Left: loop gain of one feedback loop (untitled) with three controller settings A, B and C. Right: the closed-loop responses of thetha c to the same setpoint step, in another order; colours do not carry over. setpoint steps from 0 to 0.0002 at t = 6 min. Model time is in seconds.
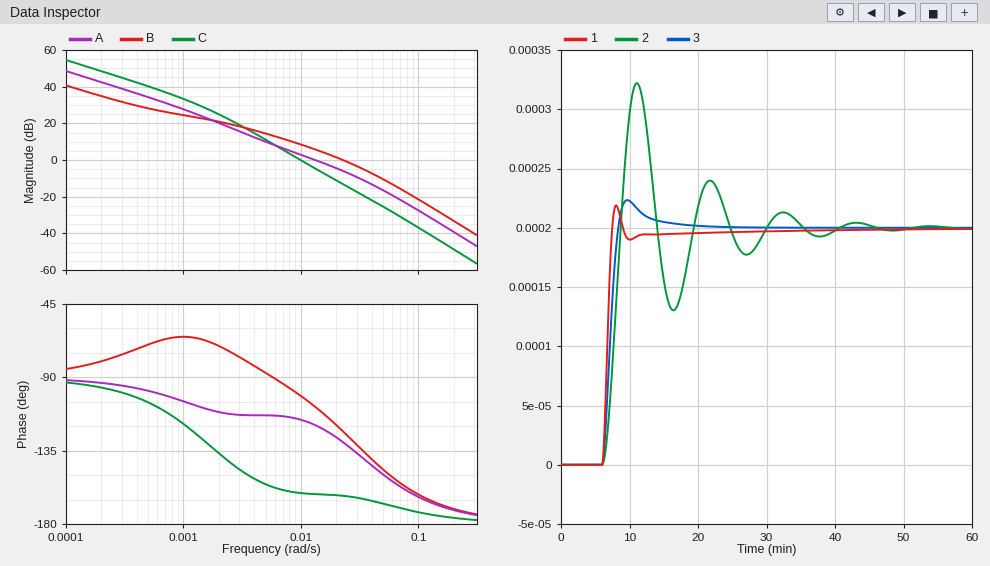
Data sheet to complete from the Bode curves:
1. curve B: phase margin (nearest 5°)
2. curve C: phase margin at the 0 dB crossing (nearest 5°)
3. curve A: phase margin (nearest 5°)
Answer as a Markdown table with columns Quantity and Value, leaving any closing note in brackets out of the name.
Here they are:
| Quantity | Value |
|---|---|
| curve B: phase margin | 55° |
| curve C: phase margin at the 0 dB crossing | 20° |
| curve A: phase margin | 60° |
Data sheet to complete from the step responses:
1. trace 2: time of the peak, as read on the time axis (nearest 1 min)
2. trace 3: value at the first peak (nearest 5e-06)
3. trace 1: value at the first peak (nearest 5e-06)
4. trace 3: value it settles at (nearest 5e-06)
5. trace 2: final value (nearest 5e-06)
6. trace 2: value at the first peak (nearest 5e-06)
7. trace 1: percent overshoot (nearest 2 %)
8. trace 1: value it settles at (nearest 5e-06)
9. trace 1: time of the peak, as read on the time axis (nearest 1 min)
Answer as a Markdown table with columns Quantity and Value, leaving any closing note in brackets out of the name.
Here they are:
| Quantity | Value |
|---|---|
| trace 2: time of the peak, as read on the time axis | 11 min |
| trace 3: value at the first peak | 0.000225 |
| trace 1: value at the first peak | 0.000220 |
| trace 3: value it settles at | 0.000200 |
| trace 2: final value | 0.000200 |
| trace 2: value at the first peak | 0.000320 |
| trace 1: percent overshoot | 10 % |
| trace 1: value it settles at | 0.000200 |
| trace 1: time of the peak, as read on the time axis | 8 min |
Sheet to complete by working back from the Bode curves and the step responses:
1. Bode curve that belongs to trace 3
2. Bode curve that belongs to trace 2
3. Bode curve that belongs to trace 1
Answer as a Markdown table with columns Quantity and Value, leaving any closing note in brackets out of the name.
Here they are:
| Quantity | Value |
|---|---|
| Bode curve that belongs to trace 3 | A |
| Bode curve that belongs to trace 2 | C |
| Bode curve that belongs to trace 1 | B |
